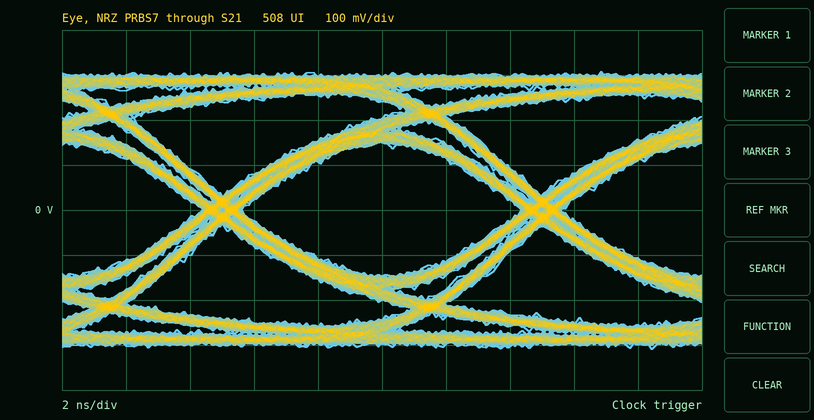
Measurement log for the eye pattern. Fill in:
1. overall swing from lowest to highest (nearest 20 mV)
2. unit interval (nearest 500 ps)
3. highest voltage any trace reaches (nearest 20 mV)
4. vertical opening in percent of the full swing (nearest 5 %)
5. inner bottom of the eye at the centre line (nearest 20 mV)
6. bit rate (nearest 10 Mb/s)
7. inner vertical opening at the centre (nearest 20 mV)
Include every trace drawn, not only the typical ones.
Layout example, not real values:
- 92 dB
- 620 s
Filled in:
- 620 mV
- 10.0 ns
- 300 mV
- 50 %
- -140 mV
- 100 Mb/s
- 300 mV
